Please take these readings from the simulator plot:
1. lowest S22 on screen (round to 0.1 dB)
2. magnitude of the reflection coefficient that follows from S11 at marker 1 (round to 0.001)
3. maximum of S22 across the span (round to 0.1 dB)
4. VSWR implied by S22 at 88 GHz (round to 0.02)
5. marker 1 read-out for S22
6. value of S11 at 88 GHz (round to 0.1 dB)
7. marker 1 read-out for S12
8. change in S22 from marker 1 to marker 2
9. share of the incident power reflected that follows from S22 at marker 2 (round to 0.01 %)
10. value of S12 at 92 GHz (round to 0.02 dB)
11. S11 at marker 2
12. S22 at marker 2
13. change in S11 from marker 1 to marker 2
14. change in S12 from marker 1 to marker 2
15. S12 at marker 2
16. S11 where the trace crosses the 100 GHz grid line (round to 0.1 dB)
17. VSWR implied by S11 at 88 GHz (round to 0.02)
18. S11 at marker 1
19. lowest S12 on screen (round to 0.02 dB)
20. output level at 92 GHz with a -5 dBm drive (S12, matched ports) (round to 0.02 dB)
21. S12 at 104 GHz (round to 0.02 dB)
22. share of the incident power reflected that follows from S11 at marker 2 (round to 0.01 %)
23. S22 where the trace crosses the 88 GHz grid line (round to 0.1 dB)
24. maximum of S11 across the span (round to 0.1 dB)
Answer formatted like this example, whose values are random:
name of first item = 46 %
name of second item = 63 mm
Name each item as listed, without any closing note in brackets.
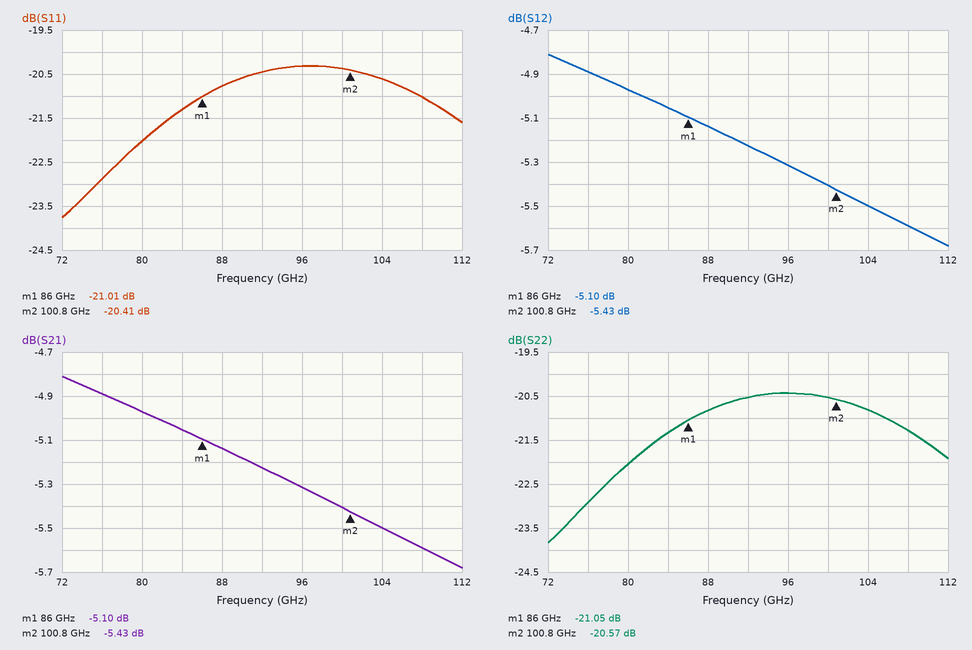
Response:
lowest S22 on screen = -23.8 dB
magnitude of the reflection coefficient that follows from S11 at marker 1 = 0.089
maximum of S22 across the span = -20.4 dB
VSWR implied by S22 at 88 GHz = 1.20
marker 1 read-out for S22 = -21.05 dB
value of S11 at 88 GHz = -20.8 dB
marker 1 read-out for S12 = -5.10 dB
change in S22 from marker 1 to marker 2 = 0.48 dB
share of the incident power reflected that follows from S22 at marker 2 = 0.88 %
value of S12 at 92 GHz = -5.22 dB
S11 at marker 2 = -20.41 dB
S22 at marker 2 = -20.57 dB
change in S11 from marker 1 to marker 2 = 0.60 dB
change in S12 from marker 1 to marker 2 = -0.33 dB
S12 at marker 2 = -5.43 dB
S11 where the trace crosses the 100 GHz grid line = -20.4 dB
VSWR implied by S11 at 88 GHz = 1.20
S11 at marker 1 = -21.01 dB
lowest S12 on screen = -5.68 dB
output level at 92 GHz with a -5 dBm drive (S12, matched ports) = -10.22 dBm
S12 at 104 GHz = -5.50 dB
share of the incident power reflected that follows from S11 at marker 2 = 0.91 %
S22 where the trace crosses the 88 GHz grid line = -20.8 dB
maximum of S11 across the span = -20.3 dB
